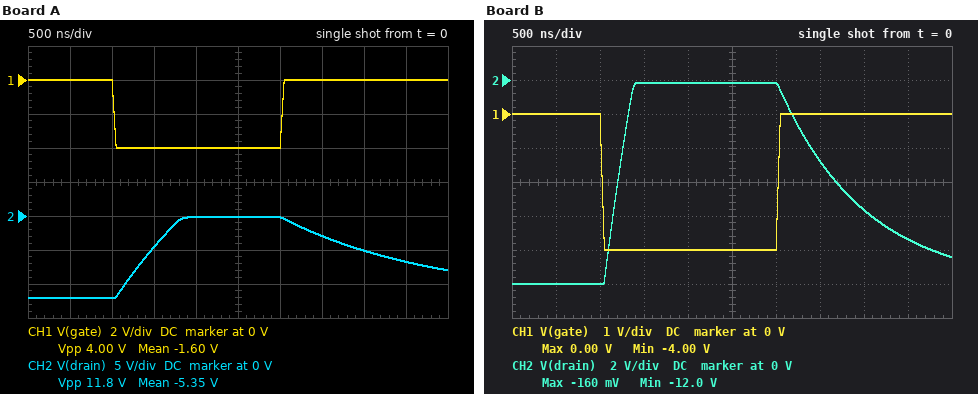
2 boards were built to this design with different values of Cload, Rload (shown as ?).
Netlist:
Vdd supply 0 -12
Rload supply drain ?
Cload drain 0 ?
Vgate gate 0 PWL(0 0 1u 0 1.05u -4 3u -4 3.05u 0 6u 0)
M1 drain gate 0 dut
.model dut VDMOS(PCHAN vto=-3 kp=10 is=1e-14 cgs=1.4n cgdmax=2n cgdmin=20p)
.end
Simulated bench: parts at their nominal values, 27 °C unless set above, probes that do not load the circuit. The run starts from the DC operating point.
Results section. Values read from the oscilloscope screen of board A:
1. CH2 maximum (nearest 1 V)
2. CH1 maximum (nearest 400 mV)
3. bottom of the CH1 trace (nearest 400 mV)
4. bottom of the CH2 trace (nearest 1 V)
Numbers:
0 V
0 V
-4.0 V
-12 V
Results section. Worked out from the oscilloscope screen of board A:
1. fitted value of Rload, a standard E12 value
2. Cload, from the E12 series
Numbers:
6.8 Ω
270 nF
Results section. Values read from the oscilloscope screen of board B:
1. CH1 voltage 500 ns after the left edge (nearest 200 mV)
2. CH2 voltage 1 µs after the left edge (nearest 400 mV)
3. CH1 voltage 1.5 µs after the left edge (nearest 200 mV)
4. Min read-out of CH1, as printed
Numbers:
0 V
-12.0 V
-4.0 V
-4.00 V
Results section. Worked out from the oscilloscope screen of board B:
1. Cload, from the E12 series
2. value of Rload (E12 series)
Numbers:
120 nF
8.2 Ω
